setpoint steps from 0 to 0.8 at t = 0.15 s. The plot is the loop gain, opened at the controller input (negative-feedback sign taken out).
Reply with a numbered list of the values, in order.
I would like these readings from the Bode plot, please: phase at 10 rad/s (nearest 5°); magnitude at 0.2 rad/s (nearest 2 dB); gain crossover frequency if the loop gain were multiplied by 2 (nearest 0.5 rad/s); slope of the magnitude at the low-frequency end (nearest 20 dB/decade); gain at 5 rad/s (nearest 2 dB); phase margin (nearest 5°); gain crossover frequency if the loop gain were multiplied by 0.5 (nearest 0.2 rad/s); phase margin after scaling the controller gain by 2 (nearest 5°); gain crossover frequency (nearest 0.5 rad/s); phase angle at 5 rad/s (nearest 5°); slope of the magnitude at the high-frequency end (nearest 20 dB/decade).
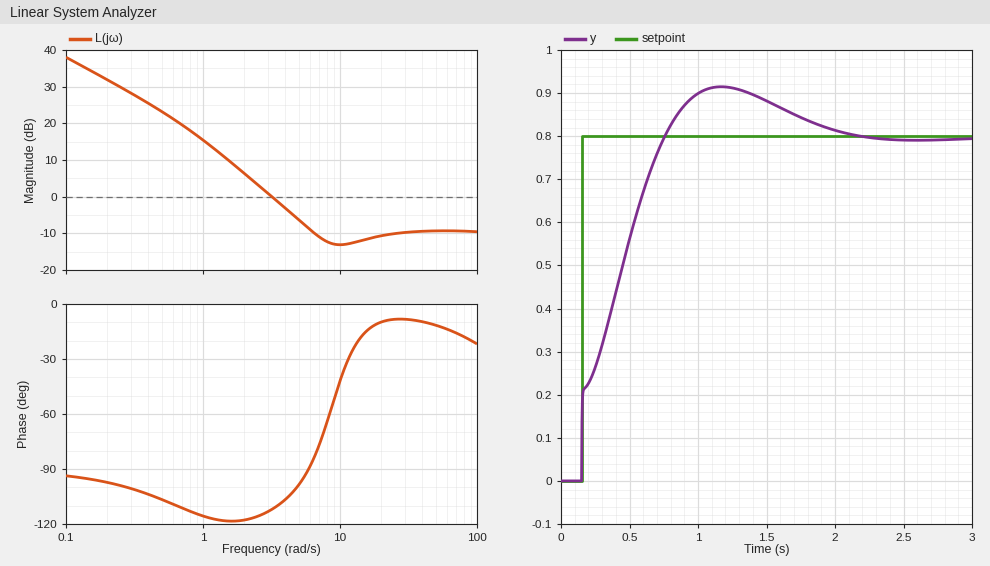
1. -40°
2. 32 dB
3. 5.0 rad/s
4. -20 dB/decade
5. -6 dB
6. 70°
7. 2.0 rad/s
8. 80°
9. 3.0 rad/s
10. -100°
11. 0 dB/decade
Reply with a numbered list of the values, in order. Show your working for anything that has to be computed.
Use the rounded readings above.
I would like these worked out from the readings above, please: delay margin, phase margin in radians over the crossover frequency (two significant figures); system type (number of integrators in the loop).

1. 70 × π / 180 / 3 = 0.41 s
2. 1
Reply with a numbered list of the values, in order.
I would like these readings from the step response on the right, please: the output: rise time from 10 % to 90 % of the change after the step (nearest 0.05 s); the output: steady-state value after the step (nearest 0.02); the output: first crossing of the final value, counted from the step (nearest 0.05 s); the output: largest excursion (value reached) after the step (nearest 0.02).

1. 0.50 s
2. 0.80
3. 0.60 s
4. 0.92
